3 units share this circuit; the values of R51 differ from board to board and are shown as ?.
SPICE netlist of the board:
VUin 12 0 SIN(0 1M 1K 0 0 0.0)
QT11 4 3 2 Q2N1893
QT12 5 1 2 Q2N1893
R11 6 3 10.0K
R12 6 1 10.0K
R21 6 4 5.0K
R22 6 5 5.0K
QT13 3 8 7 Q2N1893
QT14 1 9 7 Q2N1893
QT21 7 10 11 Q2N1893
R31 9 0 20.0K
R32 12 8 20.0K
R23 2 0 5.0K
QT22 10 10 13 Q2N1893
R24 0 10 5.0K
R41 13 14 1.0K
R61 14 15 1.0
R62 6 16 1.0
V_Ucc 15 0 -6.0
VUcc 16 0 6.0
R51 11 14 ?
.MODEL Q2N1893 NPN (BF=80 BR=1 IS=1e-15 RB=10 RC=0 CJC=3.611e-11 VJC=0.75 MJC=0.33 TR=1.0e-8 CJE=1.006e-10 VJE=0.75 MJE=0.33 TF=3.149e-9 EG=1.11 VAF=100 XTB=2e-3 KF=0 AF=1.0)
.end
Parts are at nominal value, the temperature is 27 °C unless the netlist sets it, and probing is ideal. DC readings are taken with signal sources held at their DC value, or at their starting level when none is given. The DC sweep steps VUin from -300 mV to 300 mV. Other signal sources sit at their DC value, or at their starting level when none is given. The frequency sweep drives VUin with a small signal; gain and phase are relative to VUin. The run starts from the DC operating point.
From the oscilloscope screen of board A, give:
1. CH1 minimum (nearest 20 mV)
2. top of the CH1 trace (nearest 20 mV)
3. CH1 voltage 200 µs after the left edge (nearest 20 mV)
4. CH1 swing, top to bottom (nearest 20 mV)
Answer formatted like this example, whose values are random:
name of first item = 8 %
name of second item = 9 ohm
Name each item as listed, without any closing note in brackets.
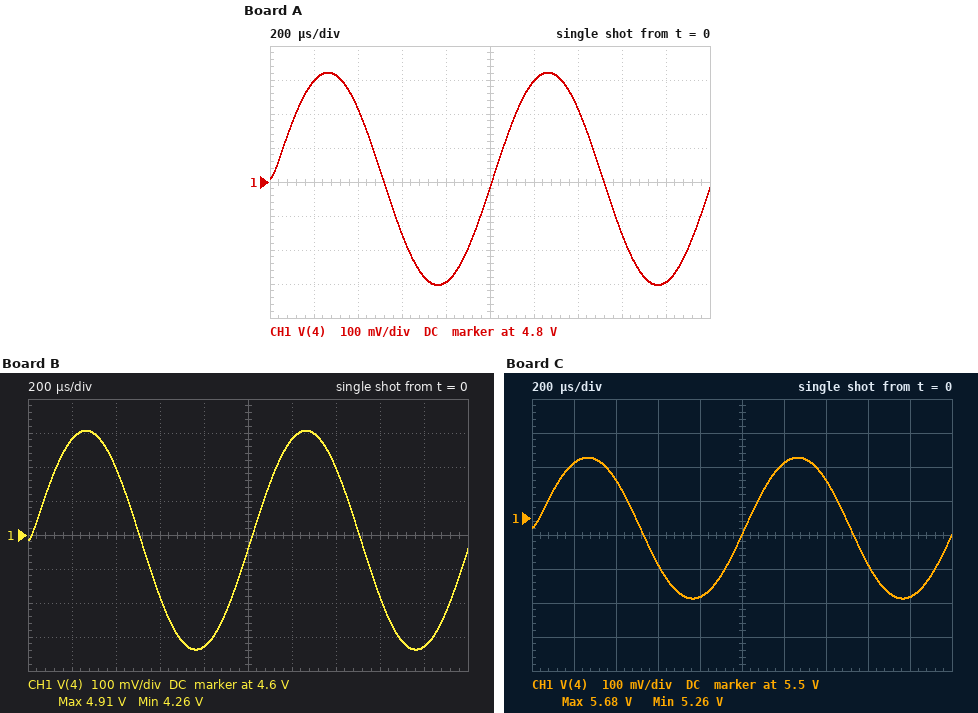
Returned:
CH1 minimum = 4.50 V
top of the CH1 trace = 5.12 V
CH1 voltage 200 µs after the left edge = 5.10 V
CH1 swing, top to bottom = 620 mV
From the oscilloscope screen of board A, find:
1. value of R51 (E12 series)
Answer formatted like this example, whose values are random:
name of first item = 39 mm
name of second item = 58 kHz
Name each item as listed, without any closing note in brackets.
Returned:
value of R51 = 1.5 kΩ
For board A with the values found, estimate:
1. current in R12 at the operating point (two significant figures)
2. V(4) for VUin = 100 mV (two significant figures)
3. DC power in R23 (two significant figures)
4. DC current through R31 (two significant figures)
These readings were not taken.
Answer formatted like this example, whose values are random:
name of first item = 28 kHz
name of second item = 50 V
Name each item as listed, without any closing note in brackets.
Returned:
current in R12 at the operating point = 290 µA
V(4) for VUin = 100 mV = 6.0 V
DC power in R23 = 1.2 mW
DC current through R31 = 3.5 µA
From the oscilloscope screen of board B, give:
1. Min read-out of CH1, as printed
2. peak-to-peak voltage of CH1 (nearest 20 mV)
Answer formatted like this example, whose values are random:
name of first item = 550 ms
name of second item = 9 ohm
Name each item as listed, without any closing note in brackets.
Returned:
Min read-out of CH1, as printed = 4.26 V
peak-to-peak voltage of CH1 = 640 mV
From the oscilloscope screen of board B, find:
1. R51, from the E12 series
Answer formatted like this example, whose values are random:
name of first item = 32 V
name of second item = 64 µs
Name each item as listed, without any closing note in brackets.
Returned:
R51, from the E12 series = 1.8 kΩ
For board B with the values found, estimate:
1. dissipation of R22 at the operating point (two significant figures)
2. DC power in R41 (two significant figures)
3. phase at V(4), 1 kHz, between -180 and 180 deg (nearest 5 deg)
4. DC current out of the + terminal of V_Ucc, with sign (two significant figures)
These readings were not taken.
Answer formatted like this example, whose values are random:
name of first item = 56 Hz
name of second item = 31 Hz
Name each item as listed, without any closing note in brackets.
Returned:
dissipation of R22 at the operating point = 400 µW
DC power in R41 = 770 µW
phase at V(4), 1 kHz, between -180 and 180 deg = -5 deg
DC current out of the + terminal of V_Ucc, with sign = -1.4 mA
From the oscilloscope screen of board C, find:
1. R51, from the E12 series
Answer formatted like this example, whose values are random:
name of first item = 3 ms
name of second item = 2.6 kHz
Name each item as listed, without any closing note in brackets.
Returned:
R51, from the E12 series = 1 kΩ
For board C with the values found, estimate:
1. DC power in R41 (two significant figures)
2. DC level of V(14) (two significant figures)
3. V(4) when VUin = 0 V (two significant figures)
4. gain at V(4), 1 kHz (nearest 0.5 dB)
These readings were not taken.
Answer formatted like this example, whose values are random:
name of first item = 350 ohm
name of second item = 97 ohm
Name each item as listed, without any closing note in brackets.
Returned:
DC power in R41 = 760 µW
DC level of V(14) = -6.0 V
V(4) when VUin = 0 V = 5.5 V
gain at V(4), 1 kHz = 46.5 dB
